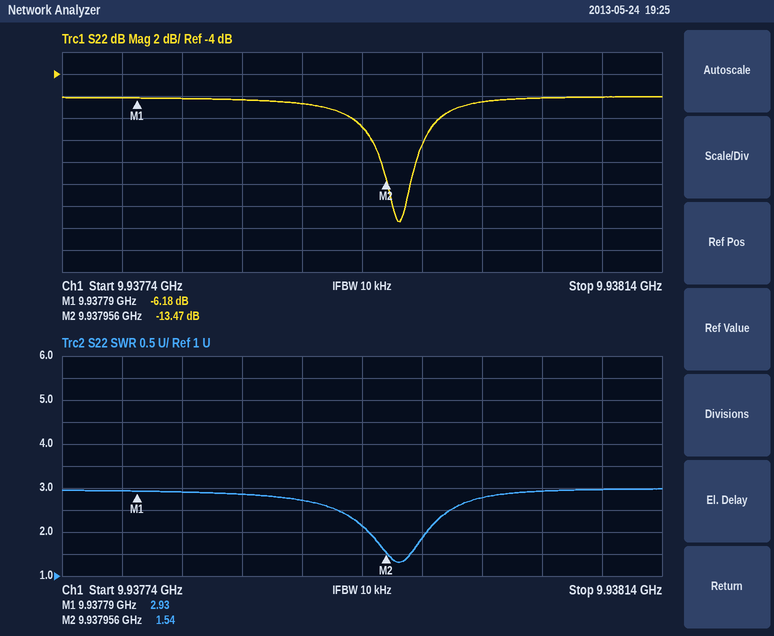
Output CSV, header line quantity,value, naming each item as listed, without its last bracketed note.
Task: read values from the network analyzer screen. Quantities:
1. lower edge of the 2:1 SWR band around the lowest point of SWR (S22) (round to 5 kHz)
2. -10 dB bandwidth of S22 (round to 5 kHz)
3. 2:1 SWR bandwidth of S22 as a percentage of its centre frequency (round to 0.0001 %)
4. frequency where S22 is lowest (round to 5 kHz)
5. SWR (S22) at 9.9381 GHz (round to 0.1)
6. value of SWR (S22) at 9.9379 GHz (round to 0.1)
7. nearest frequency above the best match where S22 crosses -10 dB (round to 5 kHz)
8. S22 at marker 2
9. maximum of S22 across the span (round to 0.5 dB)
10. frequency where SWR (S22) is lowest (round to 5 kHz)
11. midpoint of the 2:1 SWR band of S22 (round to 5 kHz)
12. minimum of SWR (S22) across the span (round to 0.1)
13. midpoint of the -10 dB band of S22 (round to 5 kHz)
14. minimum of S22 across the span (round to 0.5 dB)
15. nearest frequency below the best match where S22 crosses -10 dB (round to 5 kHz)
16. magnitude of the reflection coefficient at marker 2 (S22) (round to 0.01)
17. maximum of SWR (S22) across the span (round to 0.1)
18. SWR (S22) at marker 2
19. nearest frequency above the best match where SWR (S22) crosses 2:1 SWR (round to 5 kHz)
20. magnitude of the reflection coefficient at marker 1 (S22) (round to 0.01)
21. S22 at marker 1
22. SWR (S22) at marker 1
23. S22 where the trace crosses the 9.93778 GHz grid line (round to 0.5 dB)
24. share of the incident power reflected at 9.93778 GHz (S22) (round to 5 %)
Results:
quantity,value
lower edge of the 2:1 SWR band around the lowest point of SWR (S22),9.937945 GHz
-10 dB bandwidth of S22,35 kHz
2:1 SWR bandwidth of S22 as a percentage of its centre frequency,0.0004 %
frequency where S22 is lowest,9.937965 GHz
SWR (S22) at 9.9381 GHz,3.0
value of SWR (S22) at 9.9379 GHz,2.7
nearest frequency above the best match where S22 crosses -10 dB,9.937980 GHz
S22 at marker 2,-13.47 dB
maximum of S22 across the span,-6.0 dB
frequency where SWR (S22) is lowest,9.937965 GHz
midpoint of the 2:1 SWR band of S22,9.937965 GHz
minimum of SWR (S22) across the span,1.3
midpoint of the -10 dB band of S22,9.937965 GHz
minimum of S22 across the span,-17.5 dB
nearest frequency below the best match where S22 crosses -10 dB,9.937945 GHz
magnitude of the reflection coefficient at marker 2 (S22),0.21
maximum of SWR (S22) across the span,3.0
SWR (S22) at marker 2,1.54
nearest frequency above the best match where SWR (S22) crosses 2:1 SWR,9.937985 GHz
magnitude of the reflection coefficient at marker 1 (S22),0.49
S22 at marker 1,-6.18 dB
SWR (S22) at marker 1,2.93
S22 where the trace crosses the 9.93778 GHz grid line,-6.0 dB
share of the incident power reflected at 9.93778 GHz (S22),25 %
